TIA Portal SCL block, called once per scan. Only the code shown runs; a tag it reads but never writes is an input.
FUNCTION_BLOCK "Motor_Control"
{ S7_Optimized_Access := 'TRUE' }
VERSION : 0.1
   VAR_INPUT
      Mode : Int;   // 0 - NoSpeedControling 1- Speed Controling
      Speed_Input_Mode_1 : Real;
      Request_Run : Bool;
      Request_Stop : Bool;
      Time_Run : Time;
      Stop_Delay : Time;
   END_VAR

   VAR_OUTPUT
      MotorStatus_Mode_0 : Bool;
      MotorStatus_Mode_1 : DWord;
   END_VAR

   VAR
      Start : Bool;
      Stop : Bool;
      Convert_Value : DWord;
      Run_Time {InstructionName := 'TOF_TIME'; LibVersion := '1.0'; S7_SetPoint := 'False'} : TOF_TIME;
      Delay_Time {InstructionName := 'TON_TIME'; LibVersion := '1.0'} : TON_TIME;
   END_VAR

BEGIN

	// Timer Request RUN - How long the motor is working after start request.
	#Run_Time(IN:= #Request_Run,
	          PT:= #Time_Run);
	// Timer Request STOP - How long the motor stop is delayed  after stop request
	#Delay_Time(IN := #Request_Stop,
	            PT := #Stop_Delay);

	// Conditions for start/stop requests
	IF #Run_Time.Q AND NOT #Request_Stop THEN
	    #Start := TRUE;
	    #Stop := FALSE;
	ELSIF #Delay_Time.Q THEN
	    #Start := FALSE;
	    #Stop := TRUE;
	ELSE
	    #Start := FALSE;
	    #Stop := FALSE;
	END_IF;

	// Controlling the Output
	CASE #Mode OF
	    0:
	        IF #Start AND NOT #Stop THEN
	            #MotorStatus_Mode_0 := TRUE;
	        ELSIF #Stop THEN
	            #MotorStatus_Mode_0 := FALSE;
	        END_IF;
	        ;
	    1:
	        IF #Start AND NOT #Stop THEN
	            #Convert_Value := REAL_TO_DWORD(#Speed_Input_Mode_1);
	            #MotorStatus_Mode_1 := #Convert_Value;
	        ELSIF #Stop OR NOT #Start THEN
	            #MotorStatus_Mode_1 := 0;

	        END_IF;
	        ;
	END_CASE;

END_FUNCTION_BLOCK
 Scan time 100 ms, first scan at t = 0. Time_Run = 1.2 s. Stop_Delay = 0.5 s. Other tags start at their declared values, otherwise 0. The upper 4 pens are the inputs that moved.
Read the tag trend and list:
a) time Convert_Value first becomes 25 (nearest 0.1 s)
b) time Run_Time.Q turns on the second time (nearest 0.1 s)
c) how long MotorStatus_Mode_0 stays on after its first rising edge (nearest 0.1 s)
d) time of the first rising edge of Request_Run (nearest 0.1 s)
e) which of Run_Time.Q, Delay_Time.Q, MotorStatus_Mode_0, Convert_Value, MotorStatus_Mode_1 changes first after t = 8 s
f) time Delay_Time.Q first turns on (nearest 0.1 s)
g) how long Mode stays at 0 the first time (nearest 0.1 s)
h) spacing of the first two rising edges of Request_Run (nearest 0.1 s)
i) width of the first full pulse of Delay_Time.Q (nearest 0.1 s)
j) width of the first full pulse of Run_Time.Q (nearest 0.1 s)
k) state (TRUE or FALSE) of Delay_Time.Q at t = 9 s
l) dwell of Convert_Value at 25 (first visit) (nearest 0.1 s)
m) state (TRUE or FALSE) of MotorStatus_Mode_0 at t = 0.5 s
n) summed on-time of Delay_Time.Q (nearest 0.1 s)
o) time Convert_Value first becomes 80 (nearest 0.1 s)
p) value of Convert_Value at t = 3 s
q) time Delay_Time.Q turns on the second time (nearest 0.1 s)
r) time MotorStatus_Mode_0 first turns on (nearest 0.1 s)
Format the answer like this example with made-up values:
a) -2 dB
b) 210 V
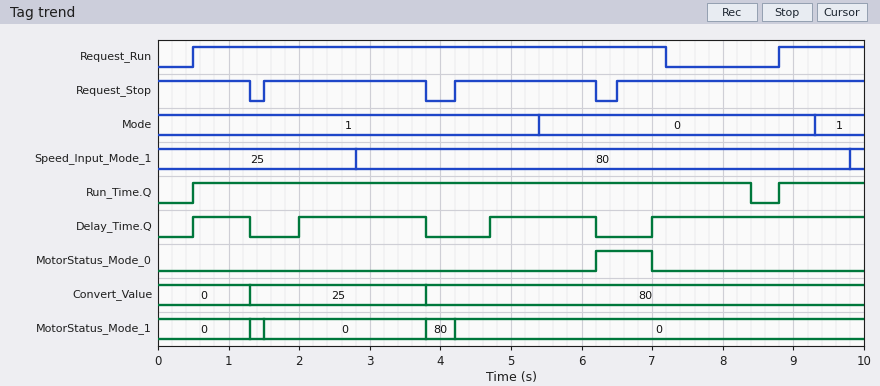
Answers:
a) 1.3 s
b) 8.8 s
c) 0.8 s
d) 0.5 s
e) Run_Time.Q
f) 0.5 s
g) 3.9 s
h) 8.3 s
i) 0.8 s
j) 7.9 s
k) TRUE
l) 2.5 s
m) FALSE
n) 7.1 s
o) 3.8 s
p) 25
q) 2.0 s
r) 6.2 s
